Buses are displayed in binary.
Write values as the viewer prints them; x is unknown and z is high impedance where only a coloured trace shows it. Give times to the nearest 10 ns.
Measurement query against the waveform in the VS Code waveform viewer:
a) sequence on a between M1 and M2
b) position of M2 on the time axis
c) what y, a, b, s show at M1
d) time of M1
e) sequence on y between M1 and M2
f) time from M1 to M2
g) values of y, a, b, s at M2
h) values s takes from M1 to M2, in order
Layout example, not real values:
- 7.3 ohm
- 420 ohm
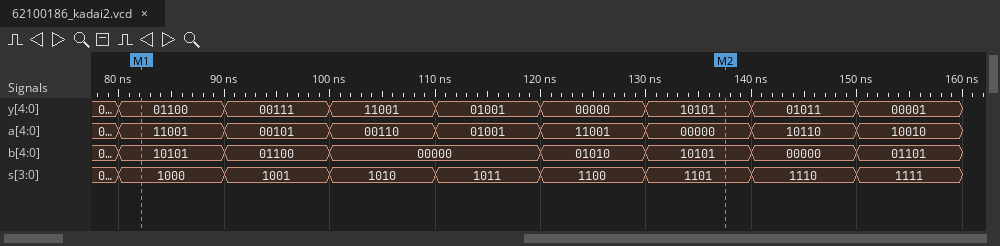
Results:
- 11001, 00101, 00110, 01001, 11001, 00000
- 140 ns
- y=01100, a=11001, b=10101, s=1000
- 80 ns
- 01100, 00111, 11001, 01001, 00000, 10101
- 60 ns
- y=10101, a=00000, b=10101, s=1101
- 1000, 1001, 1010, 1011, 1100, 1101
